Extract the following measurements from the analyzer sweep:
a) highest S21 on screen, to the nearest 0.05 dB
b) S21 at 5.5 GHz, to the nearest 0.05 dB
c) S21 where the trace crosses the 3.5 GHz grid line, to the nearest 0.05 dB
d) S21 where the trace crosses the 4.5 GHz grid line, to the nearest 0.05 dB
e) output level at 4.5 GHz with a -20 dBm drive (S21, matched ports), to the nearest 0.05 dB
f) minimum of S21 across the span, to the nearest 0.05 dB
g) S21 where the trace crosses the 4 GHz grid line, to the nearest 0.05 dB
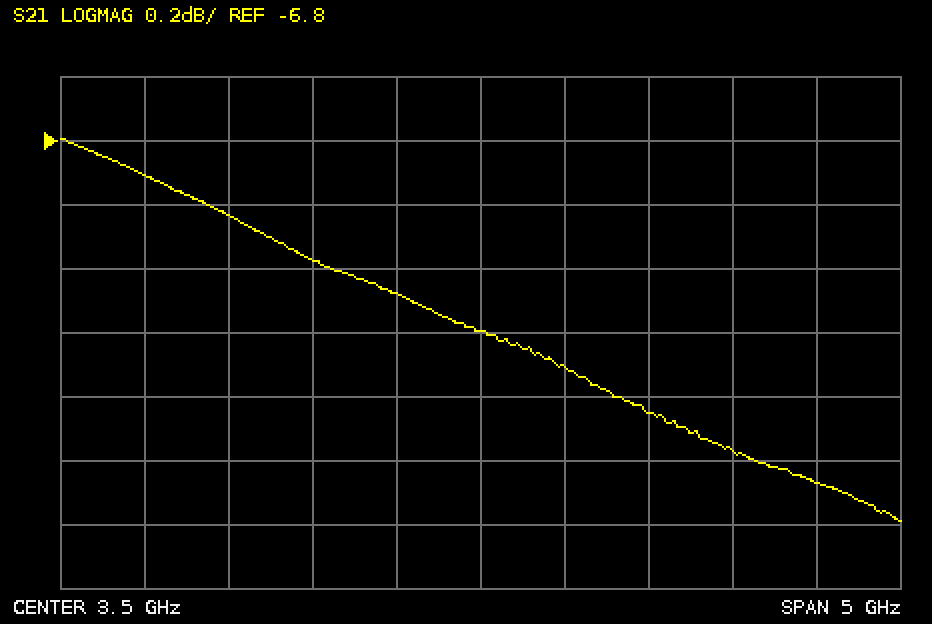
-6.80 dB
-7.85 dB
-7.40 dB
-7.65 dB
-27.65 dBm
-8.00 dB
-7.50 dB
